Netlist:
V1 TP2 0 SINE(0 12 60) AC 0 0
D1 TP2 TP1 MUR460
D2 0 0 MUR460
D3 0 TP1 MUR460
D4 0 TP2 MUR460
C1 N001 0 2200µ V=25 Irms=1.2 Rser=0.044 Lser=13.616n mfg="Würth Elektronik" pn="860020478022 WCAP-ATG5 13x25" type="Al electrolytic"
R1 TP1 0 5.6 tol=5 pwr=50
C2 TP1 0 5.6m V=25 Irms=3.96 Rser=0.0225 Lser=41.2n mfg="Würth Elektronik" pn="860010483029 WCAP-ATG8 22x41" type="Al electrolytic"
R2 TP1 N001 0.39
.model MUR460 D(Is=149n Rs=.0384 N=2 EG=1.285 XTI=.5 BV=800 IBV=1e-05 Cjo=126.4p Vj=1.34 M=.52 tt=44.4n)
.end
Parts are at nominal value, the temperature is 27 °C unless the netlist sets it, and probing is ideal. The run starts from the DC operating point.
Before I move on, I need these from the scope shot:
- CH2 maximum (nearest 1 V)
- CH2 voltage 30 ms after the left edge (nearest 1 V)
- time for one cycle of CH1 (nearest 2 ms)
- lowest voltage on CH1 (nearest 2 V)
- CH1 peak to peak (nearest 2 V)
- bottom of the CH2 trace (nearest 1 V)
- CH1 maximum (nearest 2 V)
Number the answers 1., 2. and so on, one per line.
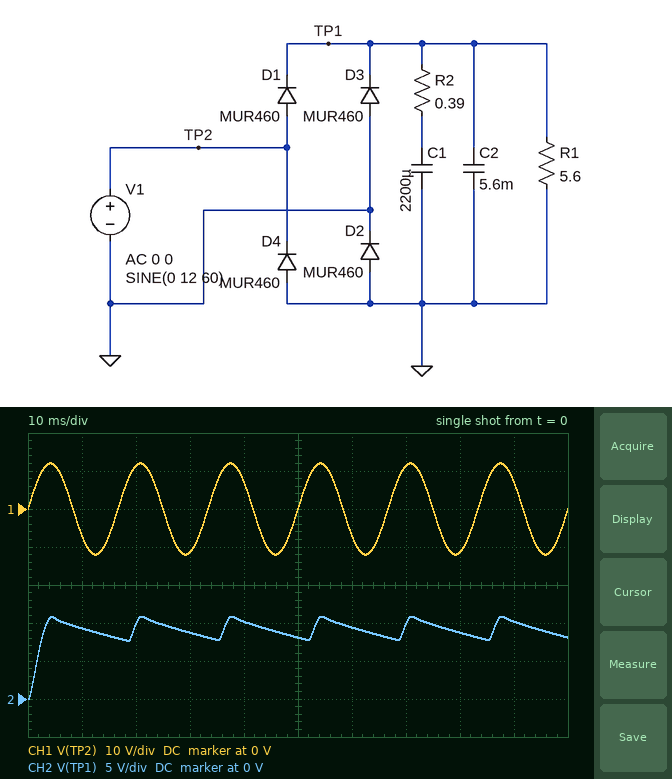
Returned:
1. 11 V
2. 9 V
3. 16 ms
4. -12 V
5. 24 V
6. 0 V
7. 12 V
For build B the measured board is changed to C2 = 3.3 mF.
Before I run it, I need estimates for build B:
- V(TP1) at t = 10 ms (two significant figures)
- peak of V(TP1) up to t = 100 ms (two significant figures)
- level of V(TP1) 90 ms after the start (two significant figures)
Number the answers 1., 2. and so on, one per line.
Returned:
1. 8.8 V
2. 11 V
3. 9.9 V
